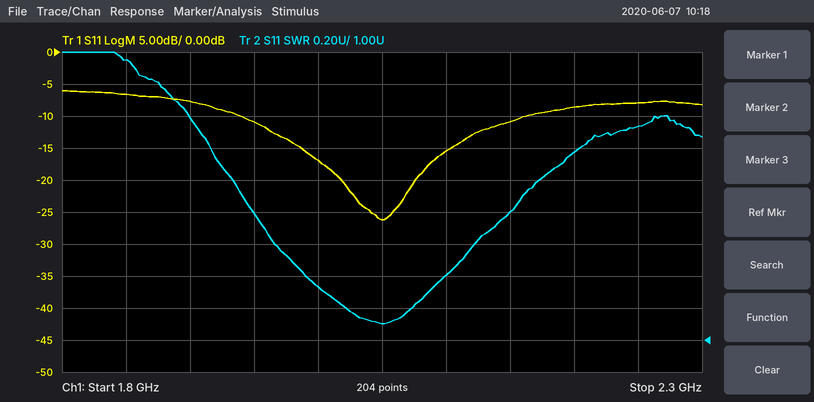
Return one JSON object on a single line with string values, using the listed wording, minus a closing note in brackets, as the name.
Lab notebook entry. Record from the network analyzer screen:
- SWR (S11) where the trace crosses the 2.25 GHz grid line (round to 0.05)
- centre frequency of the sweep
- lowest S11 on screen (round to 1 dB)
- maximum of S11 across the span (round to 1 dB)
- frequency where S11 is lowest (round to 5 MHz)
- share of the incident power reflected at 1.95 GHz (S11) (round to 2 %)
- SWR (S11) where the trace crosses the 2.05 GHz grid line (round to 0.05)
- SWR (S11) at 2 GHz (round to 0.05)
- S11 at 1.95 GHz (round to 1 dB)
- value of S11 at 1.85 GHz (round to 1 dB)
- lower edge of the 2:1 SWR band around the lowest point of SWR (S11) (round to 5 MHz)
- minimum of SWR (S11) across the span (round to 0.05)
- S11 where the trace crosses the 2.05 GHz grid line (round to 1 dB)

{"SWR (S11) where the trace crosses the 2.25 GHz grid line": "2.35", "centre frequency of the sweep": "2.05 GHz", "lowest S11 on screen": "-26 dB", "maximum of S11 across the span": "-6 dB", "frequency where S11 is lowest": "2.050 GHz", "share of the incident power reflected at 1.95 GHz (S11)": "8 %", "SWR (S11) where the trace crosses the 2.05 GHz grid line": "1.10", "SWR (S11) at 2 GHz": "1.35", "S11 at 1.95 GHz": "-11 dB", "value of S11 at 1.85 GHz": "-7 dB", "lower edge of the 2:1 SWR band around the lowest point of SWR (S11)": "1.935 GHz", "minimum of SWR (S11) across the span": "1.10", "S11 where the trace crosses the 2.05 GHz grid line": "-26 dB"}
